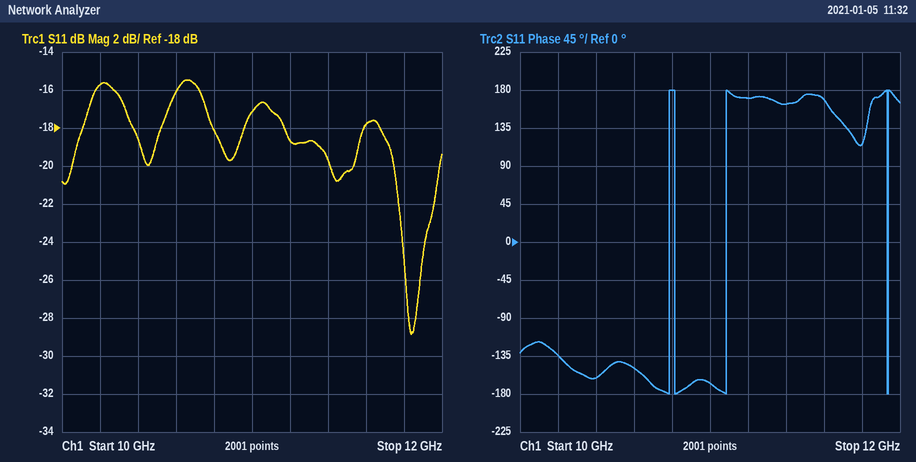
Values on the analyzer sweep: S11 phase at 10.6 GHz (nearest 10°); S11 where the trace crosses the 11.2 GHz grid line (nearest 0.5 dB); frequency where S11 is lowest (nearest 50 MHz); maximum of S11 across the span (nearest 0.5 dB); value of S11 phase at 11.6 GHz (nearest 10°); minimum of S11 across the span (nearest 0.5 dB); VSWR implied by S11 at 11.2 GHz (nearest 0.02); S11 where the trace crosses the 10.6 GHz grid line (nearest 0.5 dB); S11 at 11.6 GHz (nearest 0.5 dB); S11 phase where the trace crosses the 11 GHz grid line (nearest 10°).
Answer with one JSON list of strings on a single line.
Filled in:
["-150°", "-18.5 dB", "11.85 GHz", "-15.5 dB", "170°", "-29.0 dB", "1.26", "-16.0 dB", "-18.0 dB", "-170°"]
